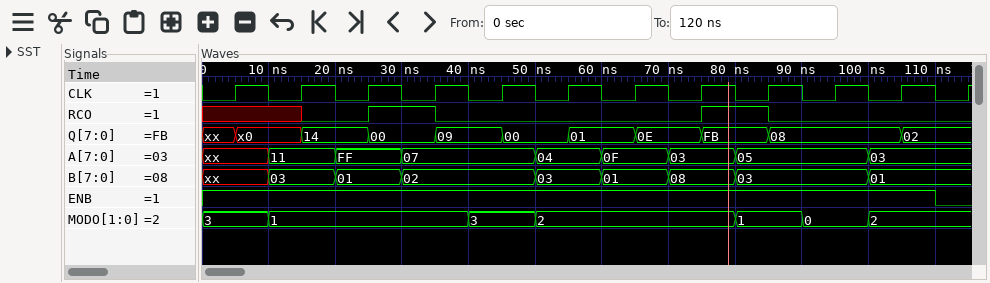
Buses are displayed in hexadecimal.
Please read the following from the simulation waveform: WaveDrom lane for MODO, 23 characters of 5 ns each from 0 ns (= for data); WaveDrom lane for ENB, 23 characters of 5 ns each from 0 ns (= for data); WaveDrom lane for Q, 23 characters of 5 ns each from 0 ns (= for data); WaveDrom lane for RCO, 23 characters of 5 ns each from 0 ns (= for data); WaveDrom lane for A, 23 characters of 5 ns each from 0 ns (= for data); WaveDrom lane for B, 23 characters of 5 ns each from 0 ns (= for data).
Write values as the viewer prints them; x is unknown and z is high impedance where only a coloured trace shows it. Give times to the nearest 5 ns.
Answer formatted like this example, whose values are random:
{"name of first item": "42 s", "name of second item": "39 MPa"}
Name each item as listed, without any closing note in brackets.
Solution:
{"WaveDrom lane for MODO, 23 characters of 5 ns each from 0 ns": "{name: 'MODO', wave: '=.=.....=.=.....=.=.=..', data: '3 1 3 2 1 0 2'}", "WaveDrom lane for ENB, 23 characters of 5 ns each from 0 ns": "{name: 'ENB', wave: '1.....................0'}", "WaveDrom lane for Q, 23 characters of 5 ns each from 0 ns": "{name: 'Q', wave: 'x=.=.=.=.=.=.=.=.=...=.', data: 'x0 14 00 09 00 01 0E FB 08 02'}", "WaveDrom lane for RCO, 23 characters of 5 ns each from 0 ns": "{name: 'RCO', wave: 'x..0.1.0.......1.0.....'}", "WaveDrom lane for A, 23 characters of 5 ns each from 0 ns": "{name: 'A', wave: 'x.=.=.=...=.=.=.=...=..', data: '11 FF 07 04 0F 03 05 03'}", "WaveDrom lane for B, 23 characters of 5 ns each from 0 ns": "{name: 'B', wave: 'x.=.=.=...=.=.=.=...=..', data: '03 01 02 03 01 08 03 01'}"}
